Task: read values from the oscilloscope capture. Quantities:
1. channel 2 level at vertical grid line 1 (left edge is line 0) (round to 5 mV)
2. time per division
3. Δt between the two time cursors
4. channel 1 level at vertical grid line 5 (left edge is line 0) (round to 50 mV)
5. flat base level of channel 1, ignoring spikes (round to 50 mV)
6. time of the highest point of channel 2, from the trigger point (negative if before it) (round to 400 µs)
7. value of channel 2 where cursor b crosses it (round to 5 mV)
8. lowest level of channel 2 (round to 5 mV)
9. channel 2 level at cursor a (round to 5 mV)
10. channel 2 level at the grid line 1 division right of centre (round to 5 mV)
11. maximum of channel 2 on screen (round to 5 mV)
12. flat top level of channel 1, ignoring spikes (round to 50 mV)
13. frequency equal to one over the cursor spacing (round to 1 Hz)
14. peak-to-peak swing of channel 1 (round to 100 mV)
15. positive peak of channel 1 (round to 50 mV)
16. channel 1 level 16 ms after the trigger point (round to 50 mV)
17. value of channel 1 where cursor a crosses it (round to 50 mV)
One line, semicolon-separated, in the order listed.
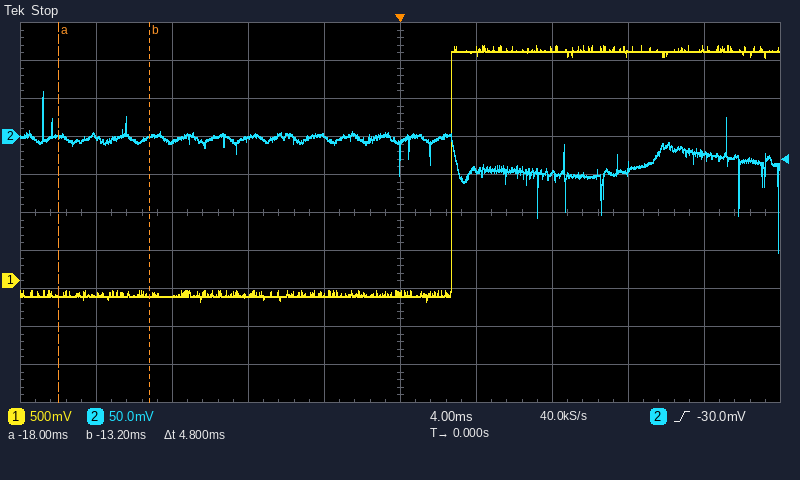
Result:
0 mV; 4 ms; 4.8 ms; -150 mV; -200 mV; -18.8 ms; 0 mV; -155 mV; 0 mV; -45 mV; 60 mV; 3.00 V; 208 Hz; 3.40 V; 3.10 V; 3.05 V; -200 mV
